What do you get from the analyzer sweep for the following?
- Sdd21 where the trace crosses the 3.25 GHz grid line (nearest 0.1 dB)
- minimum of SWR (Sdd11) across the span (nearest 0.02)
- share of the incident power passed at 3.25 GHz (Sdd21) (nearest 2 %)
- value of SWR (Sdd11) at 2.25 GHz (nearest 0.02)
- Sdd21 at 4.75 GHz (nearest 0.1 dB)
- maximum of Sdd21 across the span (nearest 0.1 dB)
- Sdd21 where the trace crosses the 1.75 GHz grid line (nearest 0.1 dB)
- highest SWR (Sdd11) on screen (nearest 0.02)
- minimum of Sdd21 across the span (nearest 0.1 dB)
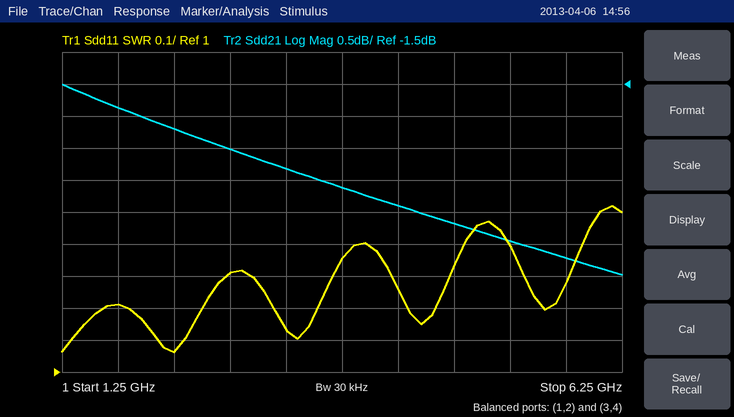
-2.8 dB
1.06
52 %
1.06
-3.7 dB
-1.5 dB
-1.9 dB
1.52
-4.5 dB
